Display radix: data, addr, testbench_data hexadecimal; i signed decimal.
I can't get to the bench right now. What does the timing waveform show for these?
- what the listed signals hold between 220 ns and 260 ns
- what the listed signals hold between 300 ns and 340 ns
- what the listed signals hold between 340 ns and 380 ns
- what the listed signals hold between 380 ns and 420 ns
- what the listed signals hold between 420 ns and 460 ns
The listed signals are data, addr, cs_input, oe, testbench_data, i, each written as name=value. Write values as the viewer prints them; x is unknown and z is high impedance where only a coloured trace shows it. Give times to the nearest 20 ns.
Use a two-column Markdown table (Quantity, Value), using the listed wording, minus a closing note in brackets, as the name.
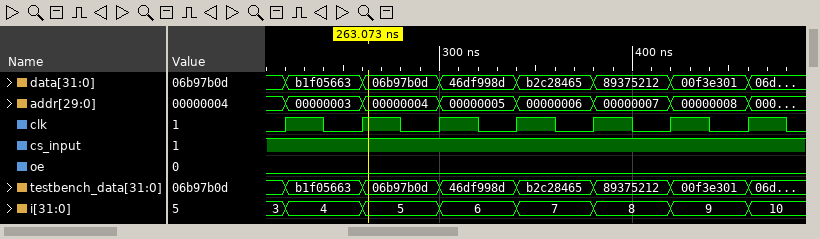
| Quantity | Value |
|---|---|
| what the listed signals hold between 220 ns and 260 ns | data=b1f05663, addr=00000003, cs_input=1, oe=0, testbench_data=b1f05663, i=4 |
| what the listed signals hold between 300 ns and 340 ns | data=46df998d, addr=00000005, cs_input=1, oe=0, testbench_data=46df998d, i=6 |
| what the listed signals hold between 340 ns and 380 ns | data=b2c28465, addr=00000006, cs_input=1, oe=0, testbench_data=b2c28465, i=7 |
| what the listed signals hold between 380 ns and 420 ns | data=89375212, addr=00000007, cs_input=1, oe=0, testbench_data=89375212, i=8 |
| what the listed signals hold between 420 ns and 460 ns | data=00f3e301, addr=00000008, cs_input=1, oe=0, testbench_data=00f3e301, i=9 |
